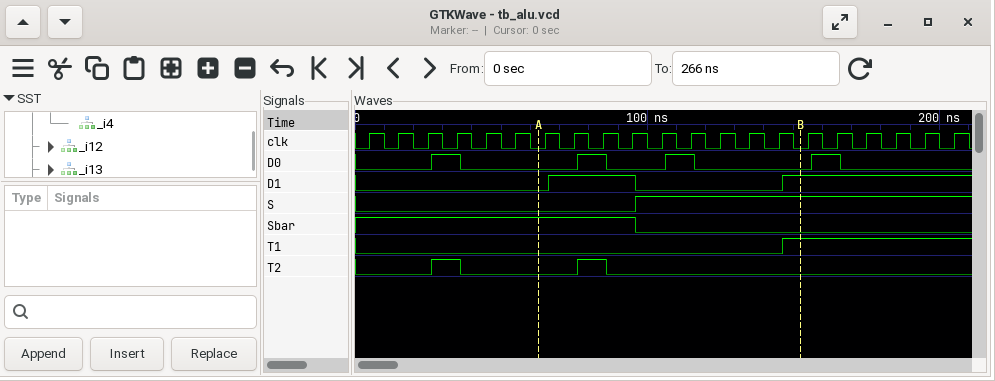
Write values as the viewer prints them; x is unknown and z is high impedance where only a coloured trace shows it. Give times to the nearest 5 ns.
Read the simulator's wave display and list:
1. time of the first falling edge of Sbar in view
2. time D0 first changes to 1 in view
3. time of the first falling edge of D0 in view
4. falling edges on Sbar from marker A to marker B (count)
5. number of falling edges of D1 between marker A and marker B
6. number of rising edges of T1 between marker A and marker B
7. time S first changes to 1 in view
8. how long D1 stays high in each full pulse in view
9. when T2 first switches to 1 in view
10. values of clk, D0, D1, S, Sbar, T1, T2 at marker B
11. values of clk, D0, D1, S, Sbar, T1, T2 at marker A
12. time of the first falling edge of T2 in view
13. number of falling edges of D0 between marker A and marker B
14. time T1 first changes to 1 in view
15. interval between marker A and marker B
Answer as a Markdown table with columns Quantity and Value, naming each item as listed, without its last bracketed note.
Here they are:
| Quantity | Value |
|---|---|
| time of the first falling edge of Sbar in view | 95 ns |
| time D0 first changes to 1 in view | 25 ns |
| time of the first falling edge of D0 in view | 35 ns |
| falling edges on Sbar from marker A to marker B | 1 |
| number of falling edges of D1 between marker A and marker B | 1 |
| number of rising edges of T1 between marker A and marker B | 1 |
| time S first changes to 1 in view | 95 ns |
| how long D1 stays high in each full pulse in view | 30 ns |
| when T2 first switches to 1 in view | 25 ns |
| values of clk, D0, D1, S, Sbar, T1, T2 at marker B | clk=0, D0=0, D1=1, S=1, Sbar=0, T1=1, T2=0 |
| values of clk, D0, D1, S, Sbar, T1, T2 at marker A | clk=0, D0=0, D1=0, S=0, Sbar=1, T1=0, T2=0 |
| time of the first falling edge of T2 in view | 35 ns |
| number of falling edges of D0 between marker A and marker B | 2 |
| time T1 first changes to 1 in view | 145 ns |
| interval between marker A and marker B | 90 ns |
